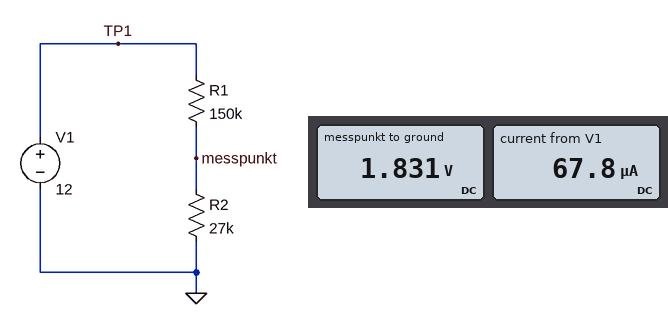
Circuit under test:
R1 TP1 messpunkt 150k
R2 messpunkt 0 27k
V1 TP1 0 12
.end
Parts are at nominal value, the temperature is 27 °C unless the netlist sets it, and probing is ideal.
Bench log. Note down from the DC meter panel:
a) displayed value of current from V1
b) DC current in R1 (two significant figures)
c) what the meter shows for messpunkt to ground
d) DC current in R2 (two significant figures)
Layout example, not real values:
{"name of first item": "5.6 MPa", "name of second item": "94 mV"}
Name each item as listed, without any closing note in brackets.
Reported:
{"displayed value of current from V1": "67.8 µA", "DC current in R1": "68 µA", "what the meter shows for messpunkt to ground": "1.831 V", "DC current in R2": "68 µA"}
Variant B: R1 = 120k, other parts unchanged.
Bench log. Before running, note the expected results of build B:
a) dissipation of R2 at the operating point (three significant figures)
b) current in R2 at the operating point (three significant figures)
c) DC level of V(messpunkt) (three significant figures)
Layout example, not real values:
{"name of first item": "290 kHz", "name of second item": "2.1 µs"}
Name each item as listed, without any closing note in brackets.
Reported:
{"dissipation of R2 at the operating point": "180 µW", "current in R2 at the operating point": "81.6 µA", "DC level of V(messpunkt)": "2.20 V"}
